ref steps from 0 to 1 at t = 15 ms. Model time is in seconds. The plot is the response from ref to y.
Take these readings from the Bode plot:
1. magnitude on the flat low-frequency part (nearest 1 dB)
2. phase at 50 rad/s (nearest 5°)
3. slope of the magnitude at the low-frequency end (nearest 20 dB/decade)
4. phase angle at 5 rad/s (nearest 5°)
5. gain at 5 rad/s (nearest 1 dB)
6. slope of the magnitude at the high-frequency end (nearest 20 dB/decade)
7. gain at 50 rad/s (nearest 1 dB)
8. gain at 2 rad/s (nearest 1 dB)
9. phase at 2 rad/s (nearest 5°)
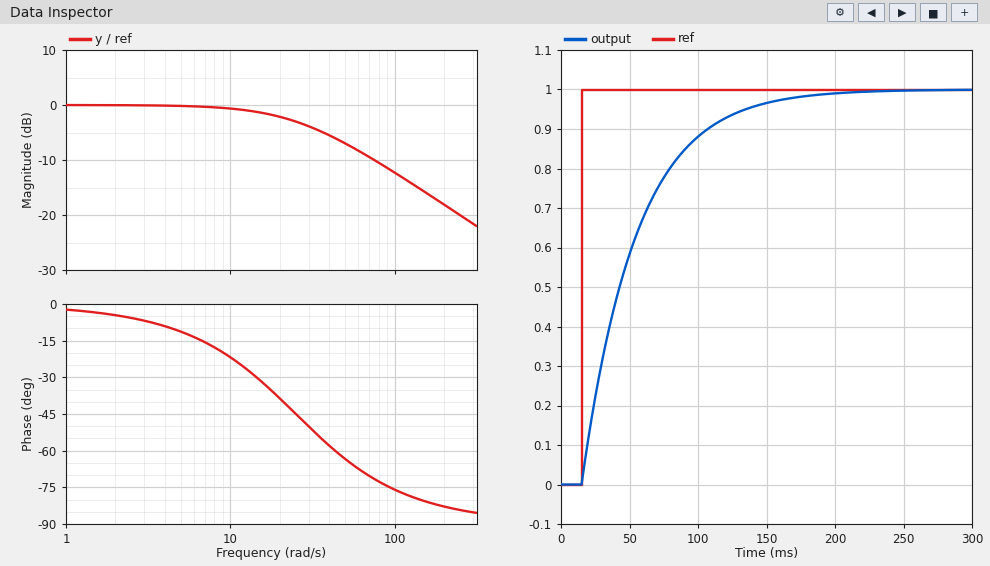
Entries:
0 dB
-65°
0 dB/decade
-10°
0 dB
-20 dB/decade
-7 dB
0 dB
-5°
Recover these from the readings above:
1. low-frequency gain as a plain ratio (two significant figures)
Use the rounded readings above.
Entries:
1.0
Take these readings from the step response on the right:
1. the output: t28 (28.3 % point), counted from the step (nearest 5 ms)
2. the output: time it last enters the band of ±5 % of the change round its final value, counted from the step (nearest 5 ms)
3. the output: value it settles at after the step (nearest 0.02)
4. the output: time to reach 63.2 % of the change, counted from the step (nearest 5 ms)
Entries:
15 ms
120 ms
1.00
40 ms
